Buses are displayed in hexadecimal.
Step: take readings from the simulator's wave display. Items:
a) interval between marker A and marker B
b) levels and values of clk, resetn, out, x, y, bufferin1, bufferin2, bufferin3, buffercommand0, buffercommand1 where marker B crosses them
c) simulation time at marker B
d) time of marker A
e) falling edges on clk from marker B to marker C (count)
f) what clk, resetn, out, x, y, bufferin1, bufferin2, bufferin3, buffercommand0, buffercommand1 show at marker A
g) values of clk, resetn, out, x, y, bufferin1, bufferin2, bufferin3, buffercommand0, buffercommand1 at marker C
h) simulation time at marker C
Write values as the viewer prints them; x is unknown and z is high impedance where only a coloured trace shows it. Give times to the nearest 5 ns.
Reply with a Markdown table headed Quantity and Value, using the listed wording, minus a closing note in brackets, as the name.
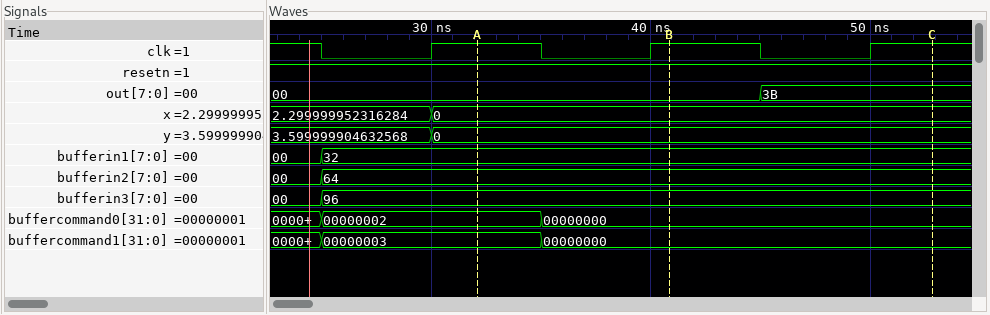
| Quantity | Value |
|---|---|
| interval between marker A and marker B | 10 ns |
| levels and values of clk, resetn, out, x, y, bufferin1, bufferin2, bufferin3, buffercommand0, buffercommand1 where marker B crosses them | clk=1, resetn=1, out=00, x=0, y=0, bufferin1=32, bufferin2=64, bufferin3=96, buffercommand0=00000000, buffercommand1=00000000 |
| simulation time at marker B | 40 ns |
| time of marker A | 30 ns |
| falling edges on clk from marker B to marker C | 1 |
| what clk, resetn, out, x, y, bufferin1, bufferin2, bufferin3, buffercommand0, buffercommand1 show at marker A | clk=1, resetn=1, out=00, x=0, y=0, bufferin1=32, bufferin2=64, bufferin3=96, buffercommand0=00000002, buffercommand1=00000003 |
| values of clk, resetn, out, x, y, bufferin1, bufferin2, bufferin3, buffercommand0, buffercommand1 at marker C | clk=1, resetn=1, out=3B, x=0, y=0, bufferin1=32, bufferin2=64, bufferin3=96, buffercommand0=00000000, buffercommand1=00000000 |
| simulation time at marker C | 55 ns |
